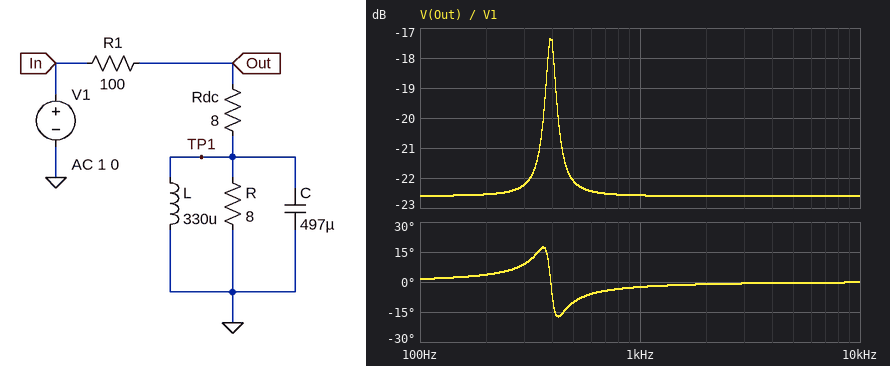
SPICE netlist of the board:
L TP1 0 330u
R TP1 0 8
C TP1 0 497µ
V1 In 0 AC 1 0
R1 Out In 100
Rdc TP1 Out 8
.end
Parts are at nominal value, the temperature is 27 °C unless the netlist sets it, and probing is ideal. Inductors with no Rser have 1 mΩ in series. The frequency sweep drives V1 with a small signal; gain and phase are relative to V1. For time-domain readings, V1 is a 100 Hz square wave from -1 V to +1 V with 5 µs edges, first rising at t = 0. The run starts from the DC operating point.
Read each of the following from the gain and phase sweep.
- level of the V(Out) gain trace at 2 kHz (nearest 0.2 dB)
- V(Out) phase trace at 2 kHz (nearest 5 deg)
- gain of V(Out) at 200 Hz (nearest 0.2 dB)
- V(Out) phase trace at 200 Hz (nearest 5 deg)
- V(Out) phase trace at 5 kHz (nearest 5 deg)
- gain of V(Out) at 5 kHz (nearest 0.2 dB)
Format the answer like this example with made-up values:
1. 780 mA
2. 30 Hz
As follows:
1. -22.6 dB
2. 0 deg
3. -22.6 dB
4. 5 deg
5. 0 deg
6. -22.6 dB
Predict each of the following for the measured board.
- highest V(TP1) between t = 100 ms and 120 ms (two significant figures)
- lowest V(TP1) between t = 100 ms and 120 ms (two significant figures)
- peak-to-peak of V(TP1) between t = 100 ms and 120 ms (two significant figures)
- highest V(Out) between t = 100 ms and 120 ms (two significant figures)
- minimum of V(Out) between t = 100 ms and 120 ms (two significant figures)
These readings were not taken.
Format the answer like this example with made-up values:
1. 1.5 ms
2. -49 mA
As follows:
1. 9.3 mV
2. -9.3 mV
3. 19 mV
4. 83 mV
5. -83 mV
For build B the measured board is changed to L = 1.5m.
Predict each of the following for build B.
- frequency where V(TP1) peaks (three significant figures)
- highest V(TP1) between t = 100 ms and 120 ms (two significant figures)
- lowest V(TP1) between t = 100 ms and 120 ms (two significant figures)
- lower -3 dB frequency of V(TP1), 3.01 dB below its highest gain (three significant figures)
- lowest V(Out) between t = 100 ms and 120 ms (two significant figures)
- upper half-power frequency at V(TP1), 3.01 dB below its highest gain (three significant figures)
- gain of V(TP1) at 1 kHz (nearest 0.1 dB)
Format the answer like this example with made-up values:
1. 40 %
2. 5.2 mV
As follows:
1. 184 Hz
2. 19 mV
3. -19 mV
4. 164 Hz
5. -92 mV
6. 207 Hz
7. -50.3 dB
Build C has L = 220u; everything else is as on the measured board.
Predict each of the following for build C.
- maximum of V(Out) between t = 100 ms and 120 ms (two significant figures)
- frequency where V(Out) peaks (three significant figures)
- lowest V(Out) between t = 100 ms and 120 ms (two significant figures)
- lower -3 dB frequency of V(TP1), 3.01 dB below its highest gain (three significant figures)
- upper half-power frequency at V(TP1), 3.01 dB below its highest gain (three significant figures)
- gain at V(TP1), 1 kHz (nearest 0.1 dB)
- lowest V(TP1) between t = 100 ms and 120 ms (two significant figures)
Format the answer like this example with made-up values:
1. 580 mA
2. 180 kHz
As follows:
1. 90 mV
2. 481 Hz
3. -90 mV
4. 460 Hz
5. 504 Hz
6. -48.3 dB
7. -17 mV
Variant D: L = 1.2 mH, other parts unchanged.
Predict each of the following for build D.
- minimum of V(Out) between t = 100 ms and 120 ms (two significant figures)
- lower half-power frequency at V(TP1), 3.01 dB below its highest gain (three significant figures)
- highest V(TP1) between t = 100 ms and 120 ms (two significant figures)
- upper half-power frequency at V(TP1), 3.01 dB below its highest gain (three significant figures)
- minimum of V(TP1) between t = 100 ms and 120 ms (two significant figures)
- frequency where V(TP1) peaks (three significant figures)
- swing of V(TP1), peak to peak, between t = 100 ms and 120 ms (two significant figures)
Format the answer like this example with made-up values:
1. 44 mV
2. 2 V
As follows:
1. -89 mV
2. 186 Hz
3. 16 mV
4. 229 Hz
5. -16 mV
6. 206 Hz
7. 33 mV
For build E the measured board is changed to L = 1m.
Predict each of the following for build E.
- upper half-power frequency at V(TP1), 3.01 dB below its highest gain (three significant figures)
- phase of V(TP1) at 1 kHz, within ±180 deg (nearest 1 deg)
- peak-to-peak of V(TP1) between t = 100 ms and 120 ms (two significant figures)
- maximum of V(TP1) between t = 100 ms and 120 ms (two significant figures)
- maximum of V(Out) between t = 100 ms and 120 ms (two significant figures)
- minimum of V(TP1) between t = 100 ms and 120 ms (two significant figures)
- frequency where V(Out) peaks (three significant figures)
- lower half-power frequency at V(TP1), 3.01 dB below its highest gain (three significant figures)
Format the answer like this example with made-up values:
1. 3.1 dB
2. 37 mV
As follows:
1. 248 Hz
2. -87 deg
3. 32 mV
4. 16 mV
5. 89 mV
6. -16 mV
7. 226 Hz
8. 205 Hz
